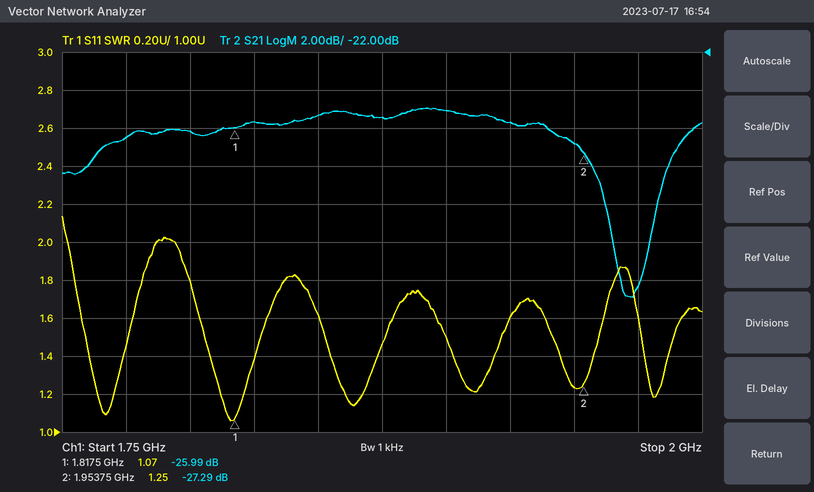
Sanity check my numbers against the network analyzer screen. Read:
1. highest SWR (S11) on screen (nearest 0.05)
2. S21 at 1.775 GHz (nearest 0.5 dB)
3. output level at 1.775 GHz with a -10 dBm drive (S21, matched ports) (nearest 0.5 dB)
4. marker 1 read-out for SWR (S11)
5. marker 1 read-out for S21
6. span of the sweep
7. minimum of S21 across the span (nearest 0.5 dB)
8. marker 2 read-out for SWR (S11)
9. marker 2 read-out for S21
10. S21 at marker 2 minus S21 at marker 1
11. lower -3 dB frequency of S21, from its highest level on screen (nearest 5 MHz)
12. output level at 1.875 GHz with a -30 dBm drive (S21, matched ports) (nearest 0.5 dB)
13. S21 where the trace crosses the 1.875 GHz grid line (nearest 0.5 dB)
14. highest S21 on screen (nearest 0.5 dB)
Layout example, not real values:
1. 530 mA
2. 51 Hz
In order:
1. 2.15
2. -26.5 dB
3. -36.5 dBm
4. 1.07
5. -25.99 dB
6. 250 MHz
7. -35.0 dB
8. 1.25
9. -27.29 dB
10. -1.30 dB
11. 1.760 GHz
12. -55.5 dBm
13. -25.5 dB
14. -25.0 dB
